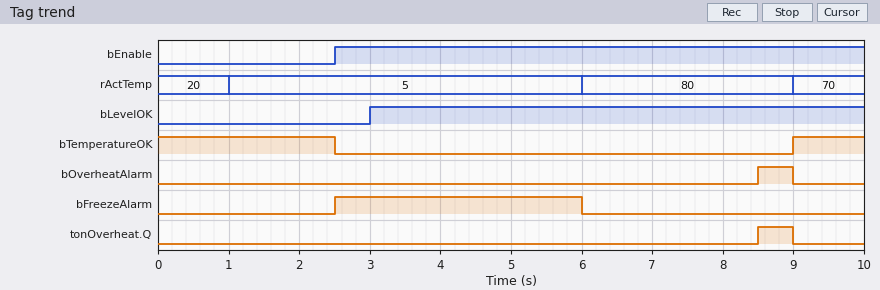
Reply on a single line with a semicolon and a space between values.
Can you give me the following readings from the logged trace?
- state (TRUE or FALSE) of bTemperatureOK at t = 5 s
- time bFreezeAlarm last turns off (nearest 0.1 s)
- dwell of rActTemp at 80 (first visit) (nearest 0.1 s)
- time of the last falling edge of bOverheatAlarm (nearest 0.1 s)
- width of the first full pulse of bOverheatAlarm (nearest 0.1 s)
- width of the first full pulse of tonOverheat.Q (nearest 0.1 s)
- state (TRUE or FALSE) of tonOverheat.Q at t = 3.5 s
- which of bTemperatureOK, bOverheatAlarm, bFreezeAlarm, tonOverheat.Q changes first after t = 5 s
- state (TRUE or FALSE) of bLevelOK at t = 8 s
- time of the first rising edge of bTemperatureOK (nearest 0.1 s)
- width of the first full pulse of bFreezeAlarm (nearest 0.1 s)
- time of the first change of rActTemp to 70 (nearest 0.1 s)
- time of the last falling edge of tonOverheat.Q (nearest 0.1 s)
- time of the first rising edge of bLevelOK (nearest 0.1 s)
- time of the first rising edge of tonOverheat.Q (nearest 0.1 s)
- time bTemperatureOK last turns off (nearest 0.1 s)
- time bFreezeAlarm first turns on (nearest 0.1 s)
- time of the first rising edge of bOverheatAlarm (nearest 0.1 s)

FALSE; 6.0 s; 3.0 s; 9.0 s; 0.5 s; 0.5 s; FALSE; bFreezeAlarm; TRUE; 9.0 s; 3.5 s; 9.0 s; 9.0 s; 3.0 s; 8.5 s; 2.5 s; 2.5 s; 8.5 s
